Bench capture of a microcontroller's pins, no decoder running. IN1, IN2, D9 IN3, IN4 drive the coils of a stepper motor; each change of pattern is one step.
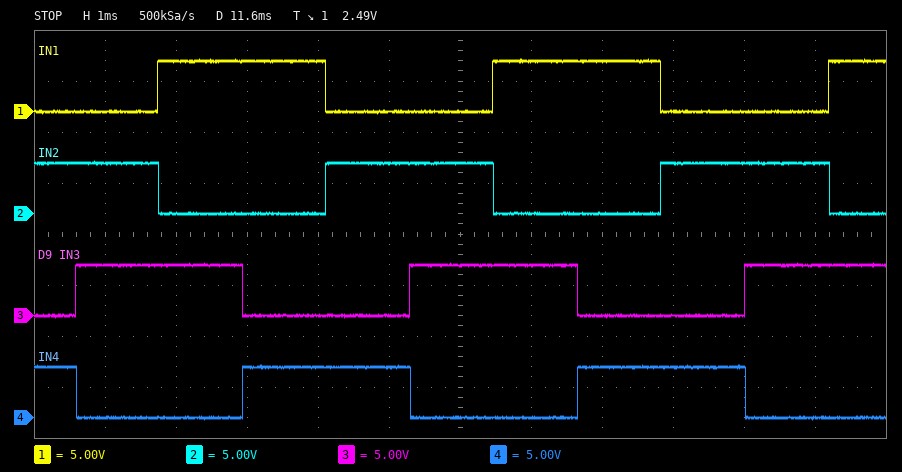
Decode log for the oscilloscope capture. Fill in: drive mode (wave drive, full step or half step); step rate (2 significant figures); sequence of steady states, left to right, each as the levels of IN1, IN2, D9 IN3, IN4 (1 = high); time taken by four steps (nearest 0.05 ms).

full step
850 steps/s
0101 0110 1010 1001 0101 0110 1010 1001 0101 0110 1010
4.70 ms
